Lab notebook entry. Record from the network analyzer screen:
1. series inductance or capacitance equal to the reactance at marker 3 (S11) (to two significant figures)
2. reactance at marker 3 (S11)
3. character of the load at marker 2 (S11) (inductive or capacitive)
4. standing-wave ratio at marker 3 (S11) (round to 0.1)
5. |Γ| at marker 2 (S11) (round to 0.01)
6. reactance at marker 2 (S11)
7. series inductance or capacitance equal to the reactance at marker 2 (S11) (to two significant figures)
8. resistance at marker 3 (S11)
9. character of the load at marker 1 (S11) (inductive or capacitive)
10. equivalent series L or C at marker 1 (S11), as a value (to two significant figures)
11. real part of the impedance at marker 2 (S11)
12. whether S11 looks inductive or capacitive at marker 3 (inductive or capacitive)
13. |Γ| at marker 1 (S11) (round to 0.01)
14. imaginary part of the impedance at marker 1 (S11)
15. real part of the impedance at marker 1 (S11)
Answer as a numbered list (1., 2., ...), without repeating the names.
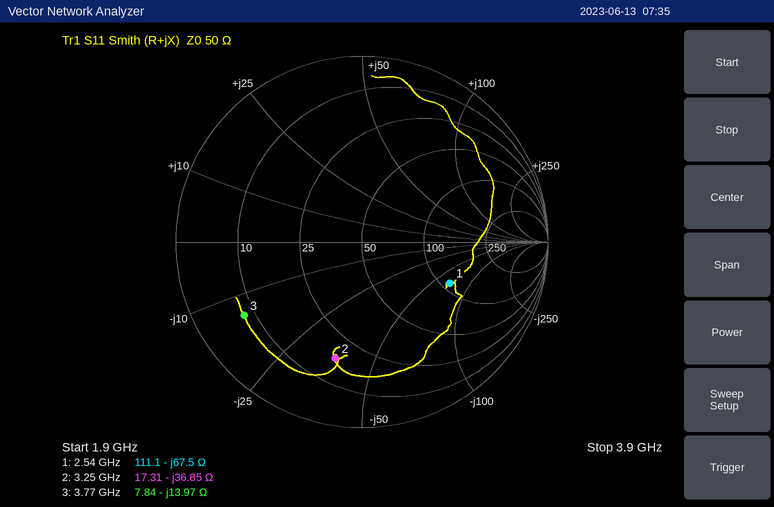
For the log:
1. 3.0 pF
2. -13.97 Ω
3. capacitive
4. 6.9
5. 0.64
6. -36.85 Ω
7. 1.3 pF
8. 7.84 Ω
9. capacitive
10. 930 fF
11. 17.31 Ω
12. capacitive
13. 0.52
14. -67.5 Ω
15. 111.1 Ω
